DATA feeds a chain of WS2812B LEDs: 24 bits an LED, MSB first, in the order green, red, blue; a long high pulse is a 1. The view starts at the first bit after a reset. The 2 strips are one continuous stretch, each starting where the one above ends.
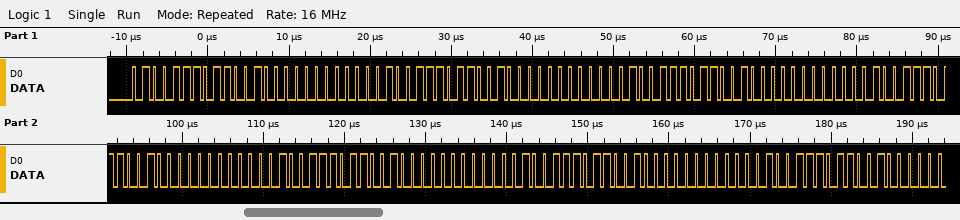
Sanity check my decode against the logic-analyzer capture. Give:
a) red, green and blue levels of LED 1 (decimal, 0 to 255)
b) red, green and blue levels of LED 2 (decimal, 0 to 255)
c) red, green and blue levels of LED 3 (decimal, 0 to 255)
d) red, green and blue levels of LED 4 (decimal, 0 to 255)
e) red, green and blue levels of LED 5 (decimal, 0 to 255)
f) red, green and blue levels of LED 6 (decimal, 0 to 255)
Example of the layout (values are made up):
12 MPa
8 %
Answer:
200, 78, 0
200, 78, 0
200, 78, 0
200, 78, 0
200, 78, 0
200, 78, 0
